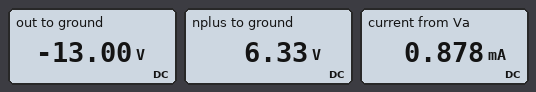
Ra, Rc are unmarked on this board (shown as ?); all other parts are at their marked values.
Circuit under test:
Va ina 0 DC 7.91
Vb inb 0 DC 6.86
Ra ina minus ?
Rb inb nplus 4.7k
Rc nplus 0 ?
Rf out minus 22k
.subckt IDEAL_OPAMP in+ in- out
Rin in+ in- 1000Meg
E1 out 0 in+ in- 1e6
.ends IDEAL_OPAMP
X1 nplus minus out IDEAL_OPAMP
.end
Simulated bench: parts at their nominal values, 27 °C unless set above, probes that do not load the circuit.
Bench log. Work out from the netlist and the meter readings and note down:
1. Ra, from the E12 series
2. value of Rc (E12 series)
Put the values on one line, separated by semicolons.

1.8 kΩ; 56 kΩ
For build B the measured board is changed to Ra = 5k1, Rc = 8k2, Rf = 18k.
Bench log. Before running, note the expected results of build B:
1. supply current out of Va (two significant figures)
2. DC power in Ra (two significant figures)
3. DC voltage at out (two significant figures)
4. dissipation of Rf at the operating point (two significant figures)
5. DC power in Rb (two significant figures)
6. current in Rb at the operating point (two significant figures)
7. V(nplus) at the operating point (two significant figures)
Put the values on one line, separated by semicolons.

700 µA; 2.5 mW; -8.2 V; 8.7 mW; 1.3 mW; 530 µA; 4.4 V
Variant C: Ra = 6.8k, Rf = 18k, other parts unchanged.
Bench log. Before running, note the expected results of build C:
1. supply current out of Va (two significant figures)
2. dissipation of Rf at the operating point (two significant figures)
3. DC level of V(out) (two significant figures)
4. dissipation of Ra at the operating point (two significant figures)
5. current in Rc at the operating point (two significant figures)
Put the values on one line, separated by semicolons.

230 µA; 970 µW; 2.1 V; 370 µW; 110 µA
